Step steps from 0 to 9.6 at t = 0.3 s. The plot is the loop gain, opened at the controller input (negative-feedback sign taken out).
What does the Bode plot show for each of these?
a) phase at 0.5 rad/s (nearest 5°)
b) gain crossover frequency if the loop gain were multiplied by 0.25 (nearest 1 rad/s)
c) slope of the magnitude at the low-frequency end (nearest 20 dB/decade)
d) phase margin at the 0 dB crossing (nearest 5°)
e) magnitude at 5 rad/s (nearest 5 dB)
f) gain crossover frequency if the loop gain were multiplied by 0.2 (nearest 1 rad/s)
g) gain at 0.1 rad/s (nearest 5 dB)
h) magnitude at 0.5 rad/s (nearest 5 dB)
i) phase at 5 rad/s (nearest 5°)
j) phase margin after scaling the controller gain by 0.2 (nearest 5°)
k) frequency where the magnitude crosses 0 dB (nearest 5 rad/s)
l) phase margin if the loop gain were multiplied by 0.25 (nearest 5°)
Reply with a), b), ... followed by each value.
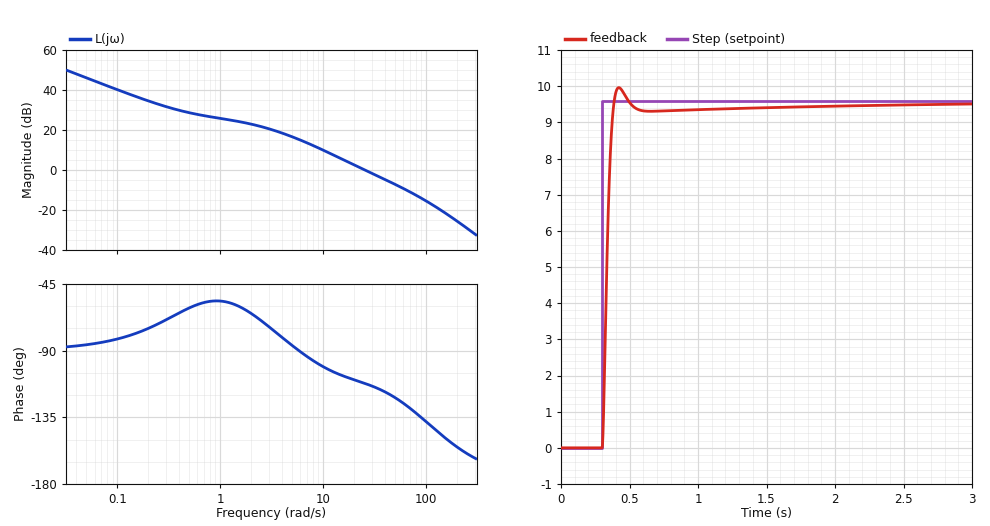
a) -60°
b) 8 rad/s
c) -20 dB/decade
d) 70°
e) 15 dB
f) 7 rad/s
g) 40 dB
h) 30 dB
i) -85°
j) 85°
k) 25 rad/s
l) 85°
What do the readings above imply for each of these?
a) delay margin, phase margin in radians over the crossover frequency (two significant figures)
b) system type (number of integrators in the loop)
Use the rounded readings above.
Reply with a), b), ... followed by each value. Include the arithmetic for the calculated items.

a) 70 × π / 180 / 25 = 0.049 s
b) 1
